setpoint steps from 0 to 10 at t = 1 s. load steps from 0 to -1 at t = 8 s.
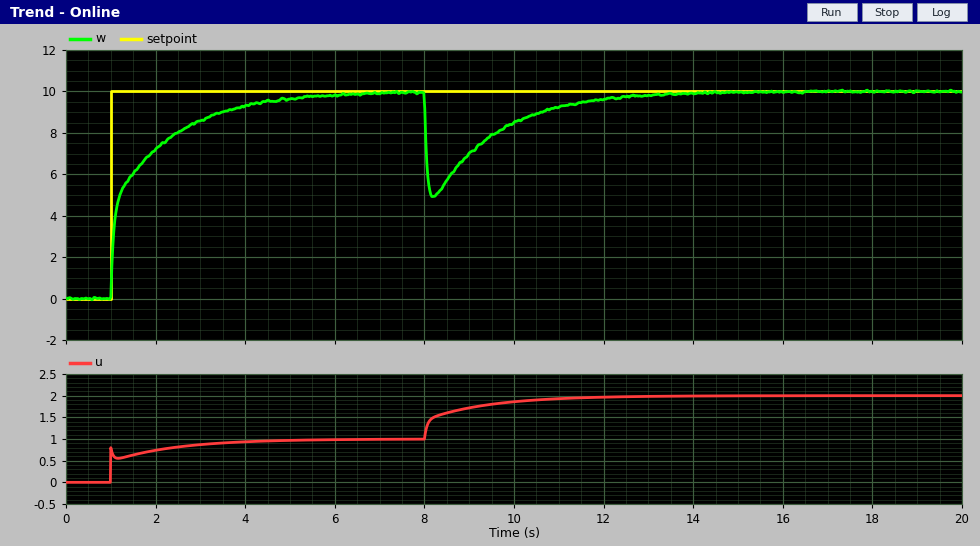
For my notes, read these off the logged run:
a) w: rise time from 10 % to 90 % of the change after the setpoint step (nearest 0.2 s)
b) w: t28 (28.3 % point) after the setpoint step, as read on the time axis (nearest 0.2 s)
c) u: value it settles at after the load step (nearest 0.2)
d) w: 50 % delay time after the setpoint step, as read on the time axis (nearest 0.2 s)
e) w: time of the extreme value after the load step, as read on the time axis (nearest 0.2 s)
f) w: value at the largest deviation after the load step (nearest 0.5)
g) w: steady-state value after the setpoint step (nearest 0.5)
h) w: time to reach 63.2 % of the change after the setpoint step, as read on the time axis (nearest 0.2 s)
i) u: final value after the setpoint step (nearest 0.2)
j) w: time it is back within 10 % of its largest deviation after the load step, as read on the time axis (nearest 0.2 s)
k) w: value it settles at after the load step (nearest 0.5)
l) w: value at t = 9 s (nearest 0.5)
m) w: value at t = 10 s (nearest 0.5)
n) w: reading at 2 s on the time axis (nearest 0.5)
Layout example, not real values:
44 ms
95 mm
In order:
2.4 s
1.0 s
2.0
1.2 s
8.2 s
5.0
10.0
1.6 s
1.0
11.6 s
10.0
7.0
8.5
7.0
